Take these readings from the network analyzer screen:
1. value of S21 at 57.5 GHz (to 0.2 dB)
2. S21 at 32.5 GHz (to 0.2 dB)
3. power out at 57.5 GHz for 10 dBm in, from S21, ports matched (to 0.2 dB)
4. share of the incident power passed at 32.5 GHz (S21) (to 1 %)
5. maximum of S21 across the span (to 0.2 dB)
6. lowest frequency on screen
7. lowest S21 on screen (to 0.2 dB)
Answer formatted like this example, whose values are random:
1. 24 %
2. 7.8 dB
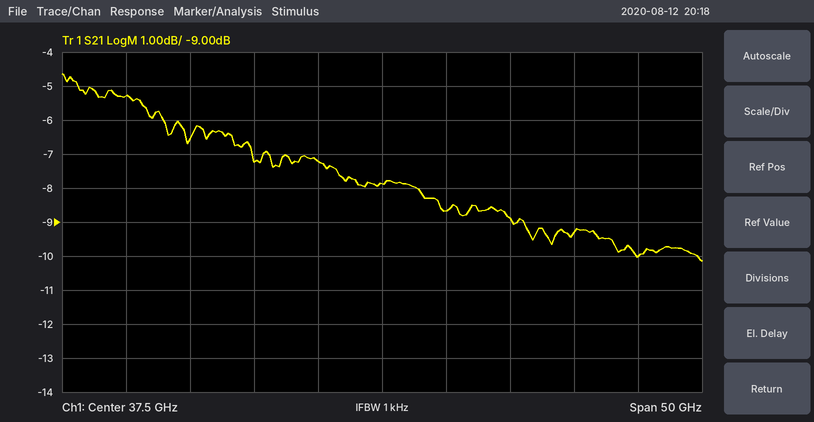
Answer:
1. -10.0 dB
2. -7.2 dB
3. 0.0 dBm
4. 19 %
5. -4.6 dB
6. 12.5 GHz
7. -10.2 dB
